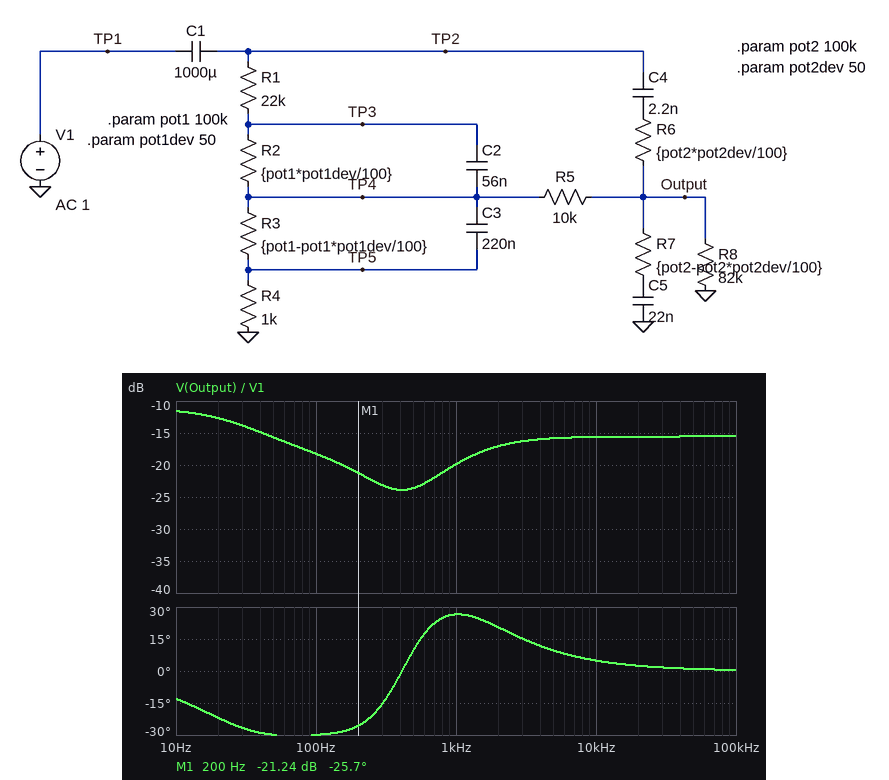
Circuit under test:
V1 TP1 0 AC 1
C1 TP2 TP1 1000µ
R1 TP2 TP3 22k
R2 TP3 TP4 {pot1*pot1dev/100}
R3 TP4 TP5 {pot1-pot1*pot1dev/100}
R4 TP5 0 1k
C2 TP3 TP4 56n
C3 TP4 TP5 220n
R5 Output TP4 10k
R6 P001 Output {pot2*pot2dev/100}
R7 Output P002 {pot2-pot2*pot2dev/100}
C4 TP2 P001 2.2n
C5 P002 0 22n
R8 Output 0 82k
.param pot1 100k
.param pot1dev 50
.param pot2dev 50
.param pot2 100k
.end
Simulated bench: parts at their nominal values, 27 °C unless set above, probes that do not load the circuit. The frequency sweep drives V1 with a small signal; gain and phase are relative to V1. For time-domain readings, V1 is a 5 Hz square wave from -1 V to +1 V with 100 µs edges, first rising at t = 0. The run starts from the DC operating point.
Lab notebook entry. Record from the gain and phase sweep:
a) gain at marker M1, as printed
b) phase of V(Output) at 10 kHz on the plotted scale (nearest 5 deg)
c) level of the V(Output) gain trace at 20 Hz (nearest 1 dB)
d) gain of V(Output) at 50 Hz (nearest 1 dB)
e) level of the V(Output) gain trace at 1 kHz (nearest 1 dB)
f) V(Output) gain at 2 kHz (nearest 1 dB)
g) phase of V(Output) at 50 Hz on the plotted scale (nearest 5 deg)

-21.24 dB
5 deg
-13 dB
-16 dB
-20 dB
-17 dB
-30 deg
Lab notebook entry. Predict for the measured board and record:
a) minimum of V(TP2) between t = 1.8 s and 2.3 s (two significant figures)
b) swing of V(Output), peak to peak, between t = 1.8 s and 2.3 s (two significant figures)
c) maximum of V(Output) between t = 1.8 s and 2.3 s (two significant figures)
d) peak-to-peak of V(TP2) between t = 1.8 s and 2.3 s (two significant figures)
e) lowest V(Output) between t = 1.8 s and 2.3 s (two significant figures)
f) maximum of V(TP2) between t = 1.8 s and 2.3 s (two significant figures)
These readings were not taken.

-21 mV
560 mV
550 mV
2.0 V
-5.8 mV
2.0 V
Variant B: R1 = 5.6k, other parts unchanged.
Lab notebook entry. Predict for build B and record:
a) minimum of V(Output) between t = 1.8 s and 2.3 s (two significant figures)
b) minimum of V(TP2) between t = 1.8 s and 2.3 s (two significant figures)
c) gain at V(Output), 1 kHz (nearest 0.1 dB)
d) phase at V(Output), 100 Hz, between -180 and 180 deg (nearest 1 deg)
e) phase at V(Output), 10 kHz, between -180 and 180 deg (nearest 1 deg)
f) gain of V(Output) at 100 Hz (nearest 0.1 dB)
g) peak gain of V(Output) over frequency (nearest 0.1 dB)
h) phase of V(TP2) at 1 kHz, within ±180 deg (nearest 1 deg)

-8.1 mV
-25 mV
-15.2 dB
-15 deg
3 deg
-15.5 dB
-9.6 dB
0 deg
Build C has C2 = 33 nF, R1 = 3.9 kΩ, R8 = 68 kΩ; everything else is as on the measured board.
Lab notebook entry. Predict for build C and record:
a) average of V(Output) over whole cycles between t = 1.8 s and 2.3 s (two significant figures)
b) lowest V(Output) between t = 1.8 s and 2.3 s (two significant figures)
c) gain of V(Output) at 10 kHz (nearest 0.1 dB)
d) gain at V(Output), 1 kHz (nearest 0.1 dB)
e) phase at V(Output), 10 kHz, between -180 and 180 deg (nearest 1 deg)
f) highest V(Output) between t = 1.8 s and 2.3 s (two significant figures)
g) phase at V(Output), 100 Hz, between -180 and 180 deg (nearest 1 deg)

310 mV
-8.1 mV
-11.6 dB
-14.7 dB
4 deg
630 mV
-21 deg
